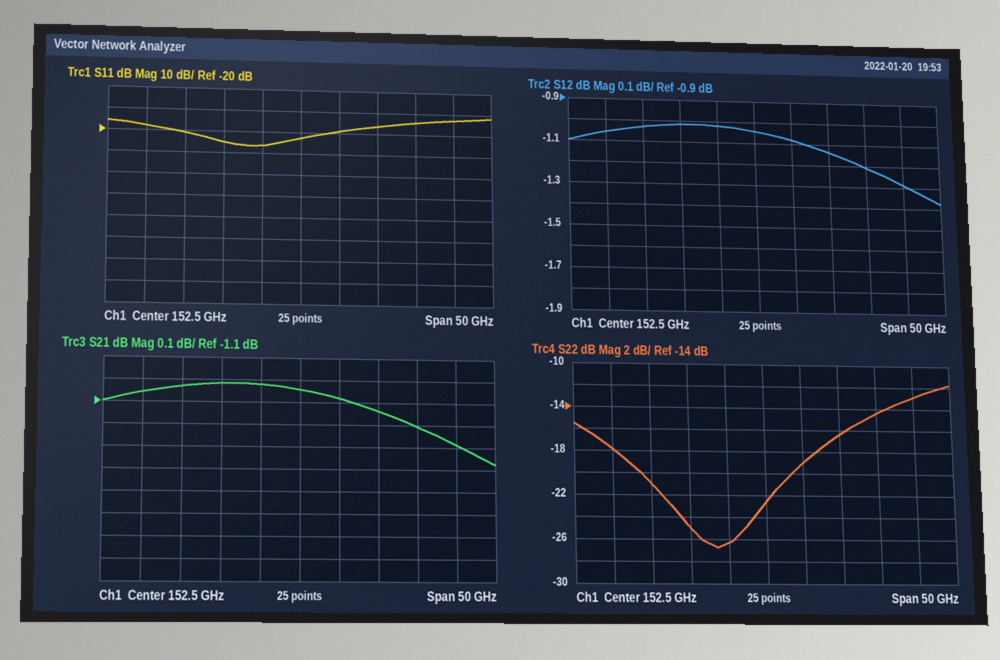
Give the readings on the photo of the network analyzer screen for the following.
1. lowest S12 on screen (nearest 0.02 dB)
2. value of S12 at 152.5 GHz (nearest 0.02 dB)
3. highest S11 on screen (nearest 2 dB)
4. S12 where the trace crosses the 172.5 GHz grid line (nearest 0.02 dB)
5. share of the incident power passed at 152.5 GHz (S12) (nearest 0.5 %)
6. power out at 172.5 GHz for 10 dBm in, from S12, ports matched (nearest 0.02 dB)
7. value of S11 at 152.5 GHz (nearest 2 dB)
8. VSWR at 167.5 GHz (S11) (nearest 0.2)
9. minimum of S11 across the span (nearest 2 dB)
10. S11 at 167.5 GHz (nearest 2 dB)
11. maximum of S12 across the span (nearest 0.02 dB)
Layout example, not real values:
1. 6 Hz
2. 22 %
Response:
1. -1.38 dB
2. -1.04 dB
3. -12 dB
4. -1.28 dB
5. 78.5 %
6. 8.72 dBm
7. -22 dB
8. 1.4
9. -26 dB
10. -14 dB
11. -1.02 dB
